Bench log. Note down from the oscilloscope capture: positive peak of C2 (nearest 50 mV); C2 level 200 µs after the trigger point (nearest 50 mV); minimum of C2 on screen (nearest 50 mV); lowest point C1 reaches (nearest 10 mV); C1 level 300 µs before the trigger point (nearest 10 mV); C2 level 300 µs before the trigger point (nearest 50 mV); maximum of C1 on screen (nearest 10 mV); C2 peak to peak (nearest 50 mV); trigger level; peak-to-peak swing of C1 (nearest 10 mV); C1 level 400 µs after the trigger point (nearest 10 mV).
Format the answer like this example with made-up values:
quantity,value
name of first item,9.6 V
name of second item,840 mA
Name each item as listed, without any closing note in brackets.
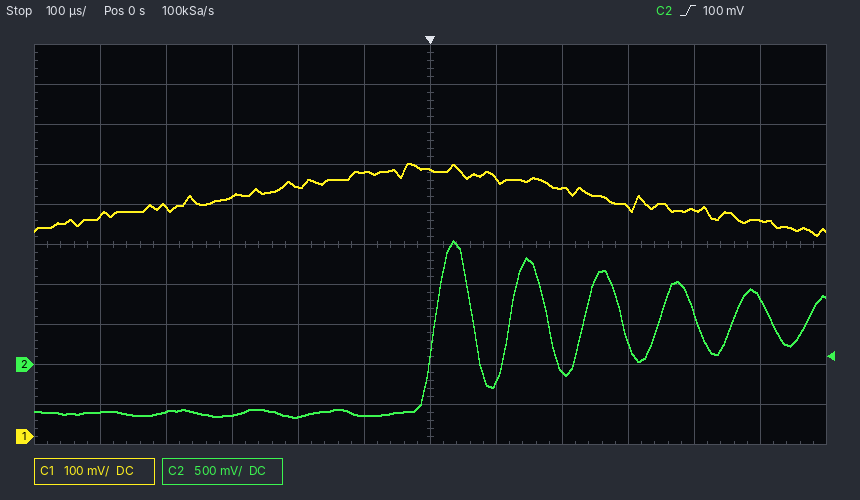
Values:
quantity,value
positive peak of C2,1.55 V
C2 level 200 µs after the trigger point,-100 mV
minimum of C2 on screen,-650 mV
lowest point C1 reaches,500 mV
C1 level 300 µs before the trigger point,600 mV
C2 level 300 µs before the trigger point,-650 mV
maximum of C1 on screen,680 mV
C2 peak to peak,2.20 V
trigger level,100 mV
peak-to-peak swing of C1,180 mV
C1 level 400 µs after the trigger point,570 mV
